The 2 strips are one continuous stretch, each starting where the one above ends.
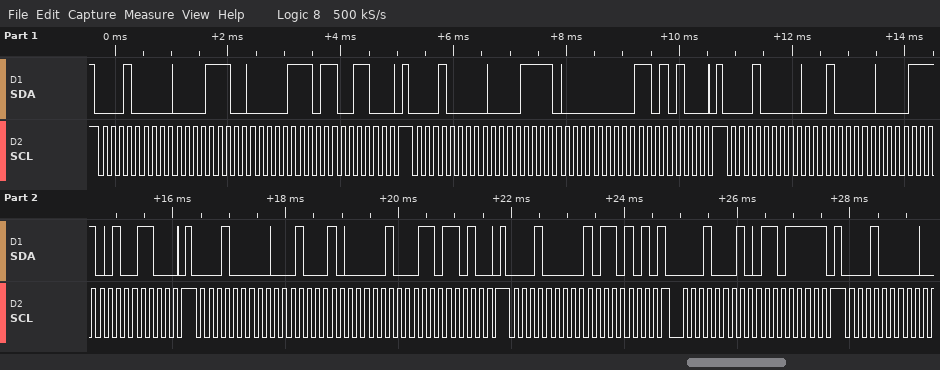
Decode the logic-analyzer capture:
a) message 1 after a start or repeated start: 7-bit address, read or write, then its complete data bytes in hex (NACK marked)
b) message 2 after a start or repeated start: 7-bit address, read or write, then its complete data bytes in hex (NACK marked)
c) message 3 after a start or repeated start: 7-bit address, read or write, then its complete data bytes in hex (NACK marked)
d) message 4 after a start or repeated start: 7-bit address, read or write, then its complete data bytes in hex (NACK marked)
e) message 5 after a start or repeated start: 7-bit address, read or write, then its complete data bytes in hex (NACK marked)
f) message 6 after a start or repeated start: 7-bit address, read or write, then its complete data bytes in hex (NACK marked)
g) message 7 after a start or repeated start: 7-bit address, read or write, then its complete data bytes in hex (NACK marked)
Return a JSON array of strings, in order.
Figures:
["0x08 write: 0E 07 CC", "0x08 write: 0F 00 D4", "0x08 write: 10 0F 4C", "0x08 write: 11 04 DA", "0x08 write: B5", "0x08 read: 6F NACK", "0x08 write"]
